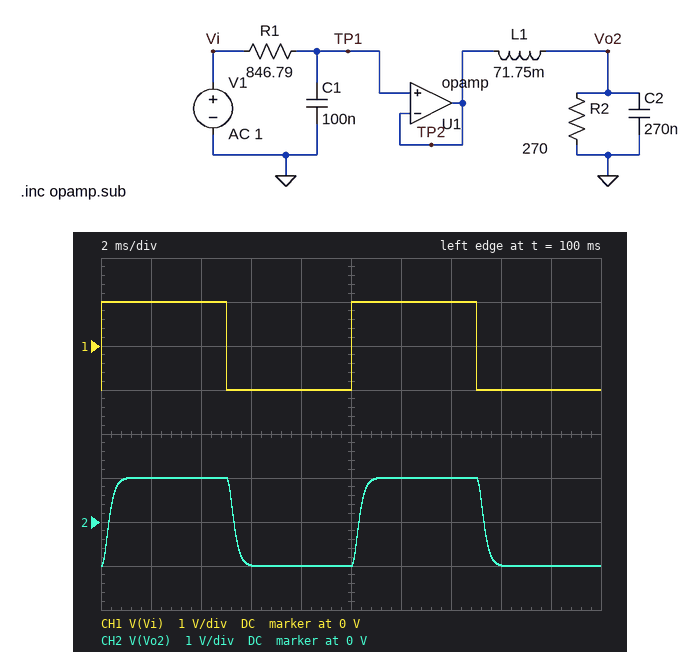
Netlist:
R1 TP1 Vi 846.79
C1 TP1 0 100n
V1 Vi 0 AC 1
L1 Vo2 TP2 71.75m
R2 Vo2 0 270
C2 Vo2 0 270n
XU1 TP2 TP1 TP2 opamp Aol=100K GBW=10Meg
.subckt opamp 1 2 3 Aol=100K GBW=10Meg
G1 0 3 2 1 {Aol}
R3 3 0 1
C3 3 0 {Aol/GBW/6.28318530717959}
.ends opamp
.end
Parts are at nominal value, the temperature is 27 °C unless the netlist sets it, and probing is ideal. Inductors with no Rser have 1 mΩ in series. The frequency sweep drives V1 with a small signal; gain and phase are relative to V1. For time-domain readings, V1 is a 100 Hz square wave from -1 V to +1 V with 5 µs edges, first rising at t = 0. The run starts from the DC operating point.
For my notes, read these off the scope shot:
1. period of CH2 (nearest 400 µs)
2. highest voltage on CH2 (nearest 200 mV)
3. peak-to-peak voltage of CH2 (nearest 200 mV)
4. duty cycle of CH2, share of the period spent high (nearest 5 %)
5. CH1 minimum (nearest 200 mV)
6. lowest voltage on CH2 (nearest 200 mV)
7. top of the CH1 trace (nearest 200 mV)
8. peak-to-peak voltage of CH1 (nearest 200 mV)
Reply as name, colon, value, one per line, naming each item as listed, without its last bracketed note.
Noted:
period of CH2: 10.0 ms
highest voltage on CH2: 1.0 V
peak-to-peak voltage of CH2: 2.0 V
duty cycle of CH2, share of the period spent high: 50 %
CH1 minimum: -1.0 V
lowest voltage on CH2: -1.0 V
top of the CH1 trace: 1.0 V
peak-to-peak voltage of CH1: 2.0 V
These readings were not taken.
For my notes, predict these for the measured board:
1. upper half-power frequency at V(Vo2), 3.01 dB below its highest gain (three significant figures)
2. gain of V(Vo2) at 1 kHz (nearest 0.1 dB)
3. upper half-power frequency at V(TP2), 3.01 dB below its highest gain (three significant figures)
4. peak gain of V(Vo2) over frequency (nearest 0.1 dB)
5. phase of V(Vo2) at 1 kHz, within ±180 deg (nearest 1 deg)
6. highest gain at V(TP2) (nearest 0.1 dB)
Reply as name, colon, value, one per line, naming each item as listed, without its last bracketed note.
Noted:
upper half-power frequency at V(Vo2), 3.01 dB below its highest gain: 700 Hz
gain of V(Vo2) at 1 kHz: -5.6 dB
upper half-power frequency at V(TP2), 3.01 dB below its highest gain: 1.88 kHz
peak gain of V(Vo2) over frequency: 0 dB
phase of V(Vo2) at 1 kHz, within ±180 deg: -110 deg
highest gain at V(TP2): 0 dB
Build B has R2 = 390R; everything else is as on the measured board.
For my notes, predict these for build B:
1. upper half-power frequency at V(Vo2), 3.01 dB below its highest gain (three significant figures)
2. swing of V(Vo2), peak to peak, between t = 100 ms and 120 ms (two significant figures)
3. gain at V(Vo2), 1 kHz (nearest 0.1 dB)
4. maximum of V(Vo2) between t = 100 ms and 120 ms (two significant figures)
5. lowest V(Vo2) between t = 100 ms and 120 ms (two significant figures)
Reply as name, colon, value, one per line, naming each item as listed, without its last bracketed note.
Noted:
upper half-power frequency at V(Vo2), 3.01 dB below its highest gain: 1.06 kHz
swing of V(Vo2), peak to peak, between t = 100 ms and 120 ms: 2.2 V
gain at V(Vo2), 1 kHz: -2.5 dB
maximum of V(Vo2) between t = 100 ms and 120 ms: 1.1 V
lowest V(Vo2) between t = 100 ms and 120 ms: -1.1 V
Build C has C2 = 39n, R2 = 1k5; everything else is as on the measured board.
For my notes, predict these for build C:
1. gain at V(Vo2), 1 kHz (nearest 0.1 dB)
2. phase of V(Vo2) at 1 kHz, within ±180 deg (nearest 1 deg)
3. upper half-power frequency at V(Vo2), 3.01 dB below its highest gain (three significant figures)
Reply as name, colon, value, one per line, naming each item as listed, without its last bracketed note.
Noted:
gain at V(Vo2), 1 kHz: -0.5 dB
phase of V(Vo2) at 1 kHz, within ±180 deg: -47 deg
upper half-power frequency at V(Vo2), 3.01 dB below its highest gain: 2.62 kHz
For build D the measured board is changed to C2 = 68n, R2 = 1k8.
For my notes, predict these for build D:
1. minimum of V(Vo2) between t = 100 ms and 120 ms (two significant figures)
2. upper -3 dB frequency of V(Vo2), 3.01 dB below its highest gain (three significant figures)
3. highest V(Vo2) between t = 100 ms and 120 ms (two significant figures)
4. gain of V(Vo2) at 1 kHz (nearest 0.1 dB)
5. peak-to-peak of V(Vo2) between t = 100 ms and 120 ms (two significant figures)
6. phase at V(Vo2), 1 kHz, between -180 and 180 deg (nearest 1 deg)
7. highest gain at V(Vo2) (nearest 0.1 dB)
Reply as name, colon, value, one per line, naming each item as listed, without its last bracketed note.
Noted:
minimum of V(Vo2) between t = 100 ms and 120 ms: -1.4 V
upper -3 dB frequency of V(Vo2), 3.01 dB below its highest gain: 2.53 kHz
highest V(Vo2) between t = 100 ms and 120 ms: 1.4 V
gain of V(Vo2) at 1 kHz: 0.4 dB
peak-to-peak of V(Vo2) between t = 100 ms and 120 ms: 2.8 V
phase at V(Vo2), 1 kHz, between -180 and 180 deg: -45 deg
highest gain at V(Vo2): 1.9 dB
